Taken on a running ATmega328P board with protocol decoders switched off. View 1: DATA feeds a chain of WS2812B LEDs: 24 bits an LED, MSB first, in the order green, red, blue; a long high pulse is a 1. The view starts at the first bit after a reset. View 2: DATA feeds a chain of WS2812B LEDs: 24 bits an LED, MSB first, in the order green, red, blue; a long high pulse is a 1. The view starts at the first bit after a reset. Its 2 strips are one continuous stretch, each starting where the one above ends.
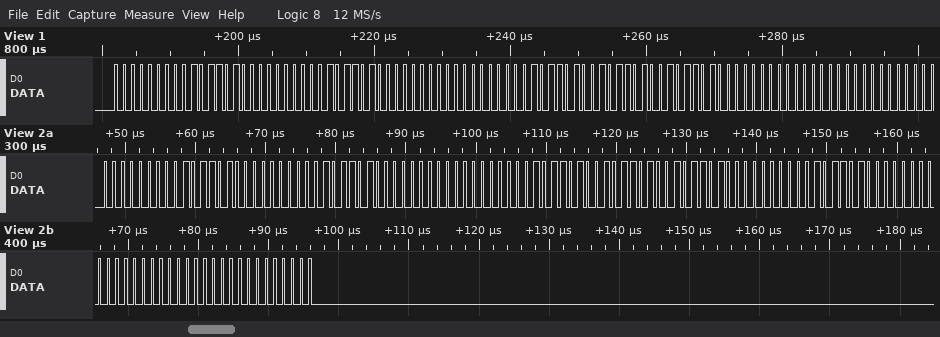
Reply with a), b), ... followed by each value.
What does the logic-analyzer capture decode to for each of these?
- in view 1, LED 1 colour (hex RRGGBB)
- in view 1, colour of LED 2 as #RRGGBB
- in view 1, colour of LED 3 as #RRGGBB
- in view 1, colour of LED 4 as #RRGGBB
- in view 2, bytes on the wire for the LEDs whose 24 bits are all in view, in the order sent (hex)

a) #5A0000
b) #005A00
c) #5A5A5A
d) #000000
e) 00 5A 00 5A 00 00 5A 5A 5A 00 5A 00 00 00 00
